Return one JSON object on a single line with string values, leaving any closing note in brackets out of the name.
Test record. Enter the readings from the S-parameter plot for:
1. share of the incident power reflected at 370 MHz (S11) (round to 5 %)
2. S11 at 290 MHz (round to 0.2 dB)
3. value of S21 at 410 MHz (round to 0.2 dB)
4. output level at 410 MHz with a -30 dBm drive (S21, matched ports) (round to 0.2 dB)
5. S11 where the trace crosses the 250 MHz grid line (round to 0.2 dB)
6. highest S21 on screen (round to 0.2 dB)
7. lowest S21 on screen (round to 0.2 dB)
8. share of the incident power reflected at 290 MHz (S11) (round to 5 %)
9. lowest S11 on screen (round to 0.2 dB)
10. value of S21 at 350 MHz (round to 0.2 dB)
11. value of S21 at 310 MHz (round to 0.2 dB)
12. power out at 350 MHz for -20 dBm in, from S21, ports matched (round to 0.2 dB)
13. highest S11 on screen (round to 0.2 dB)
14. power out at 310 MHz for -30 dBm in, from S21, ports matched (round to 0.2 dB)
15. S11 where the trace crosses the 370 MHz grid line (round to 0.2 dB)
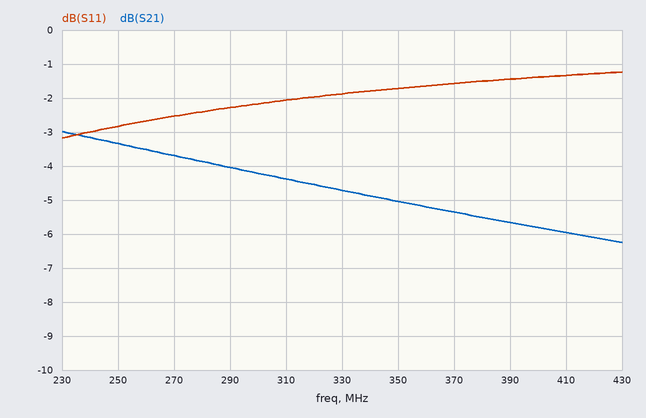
{"share of the incident power reflected at 370 MHz (S11)": "70 %", "S11 at 290 MHz": "-2.2 dB", "value of S21 at 410 MHz": "-6.0 dB", "output level at 410 MHz with a -30 dBm drive (S21, matched ports)": "-36.0 dBm", "S11 where the trace crosses the 250 MHz grid line": "-2.8 dB", "highest S21 on screen": "-3.0 dB", "lowest S21 on screen": "-6.2 dB", "share of the incident power reflected at 290 MHz (S11)": "60 %", "lowest S11 on screen": "-3.2 dB", "value of S21 at 350 MHz": "-5.0 dB", "value of S21 at 310 MHz": "-4.4 dB", "power out at 350 MHz for -20 dBm in, from S21, ports matched": "-25.0 dBm", "highest S11 on screen": "-1.2 dB", "power out at 310 MHz for -30 dBm in, from S21, ports matched": "-34.4 dBm", "S11 where the trace crosses the 370 MHz grid line": "-1.6 dB"}
